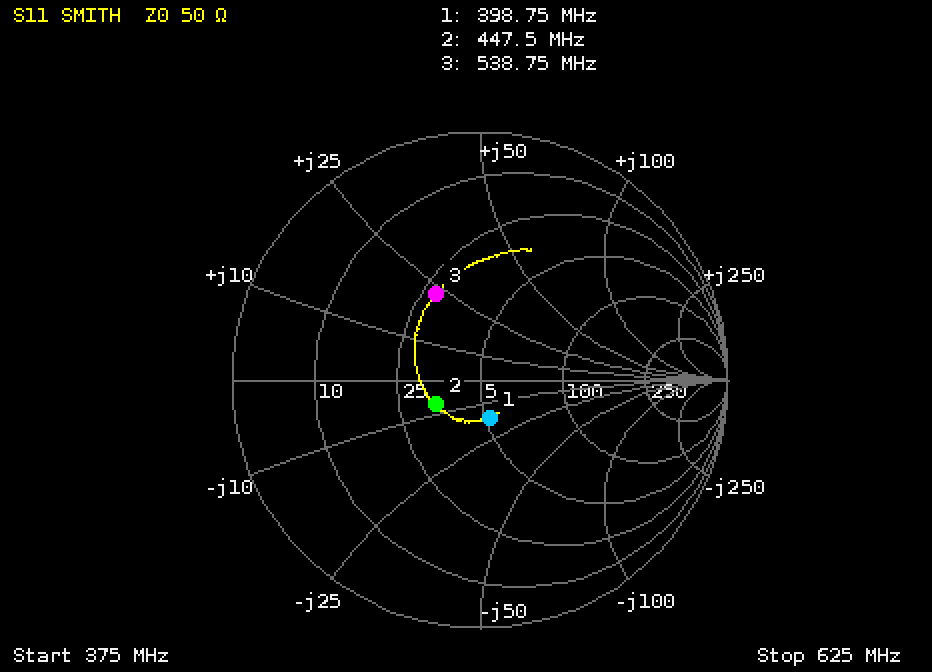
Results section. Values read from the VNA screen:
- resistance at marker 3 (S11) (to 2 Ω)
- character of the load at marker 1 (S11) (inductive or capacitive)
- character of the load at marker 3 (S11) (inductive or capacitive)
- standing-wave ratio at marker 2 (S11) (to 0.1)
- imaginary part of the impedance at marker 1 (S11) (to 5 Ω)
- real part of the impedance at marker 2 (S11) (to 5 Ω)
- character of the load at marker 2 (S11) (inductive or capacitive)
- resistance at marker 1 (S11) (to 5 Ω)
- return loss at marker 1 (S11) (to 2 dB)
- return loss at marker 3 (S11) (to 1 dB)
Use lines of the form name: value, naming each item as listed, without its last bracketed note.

resistance at marker 3 (S11): 28 Ω
character of the load at marker 1 (S11): capacitive
character of the load at marker 3 (S11): inductive
standing-wave ratio at marker 2 (S11): 1.5
imaginary part of the impedance at marker 1 (S11): -15 Ω
real part of the impedance at marker 2 (S11): 35 Ω
character of the load at marker 2 (S11): capacitive
resistance at marker 1 (S11): 50 Ω
return loss at marker 1 (S11): 16 dB
return loss at marker 3 (S11): 8 dB
